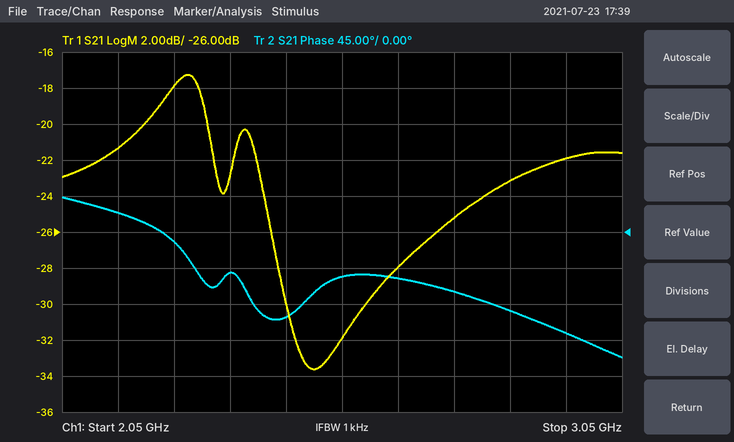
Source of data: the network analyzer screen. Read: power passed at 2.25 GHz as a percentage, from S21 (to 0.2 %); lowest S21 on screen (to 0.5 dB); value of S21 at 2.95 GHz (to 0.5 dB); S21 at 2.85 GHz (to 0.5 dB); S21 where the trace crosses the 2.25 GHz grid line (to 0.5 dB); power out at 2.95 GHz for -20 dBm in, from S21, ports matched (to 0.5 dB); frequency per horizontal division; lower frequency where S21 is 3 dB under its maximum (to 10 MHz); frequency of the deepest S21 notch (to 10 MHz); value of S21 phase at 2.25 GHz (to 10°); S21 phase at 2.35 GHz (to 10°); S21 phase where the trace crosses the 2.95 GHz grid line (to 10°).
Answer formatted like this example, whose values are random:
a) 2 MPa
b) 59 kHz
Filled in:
a) 1.6 %
b) -33.5 dB
c) -22.0 dB
d) -23.0 dB
e) -18.0 dB
f) -42.0 dBm
g) 100 MHz
h) 2.19 GHz
i) 2.50 GHz
j) -10°
k) -50°
l) -130°
